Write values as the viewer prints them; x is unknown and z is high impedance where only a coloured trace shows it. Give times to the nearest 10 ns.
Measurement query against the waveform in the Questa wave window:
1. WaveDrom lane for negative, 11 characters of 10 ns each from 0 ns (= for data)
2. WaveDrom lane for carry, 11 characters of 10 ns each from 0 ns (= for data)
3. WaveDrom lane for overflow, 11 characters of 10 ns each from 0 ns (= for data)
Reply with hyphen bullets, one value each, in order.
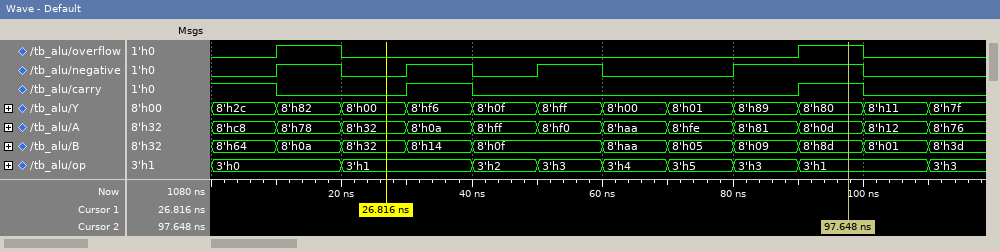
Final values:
- {name: 'negative', wave: '0101010.1.0'}
- {name: 'carry', wave: '10.10....10'}
- {name: 'overflow', wave: '010......10'}
